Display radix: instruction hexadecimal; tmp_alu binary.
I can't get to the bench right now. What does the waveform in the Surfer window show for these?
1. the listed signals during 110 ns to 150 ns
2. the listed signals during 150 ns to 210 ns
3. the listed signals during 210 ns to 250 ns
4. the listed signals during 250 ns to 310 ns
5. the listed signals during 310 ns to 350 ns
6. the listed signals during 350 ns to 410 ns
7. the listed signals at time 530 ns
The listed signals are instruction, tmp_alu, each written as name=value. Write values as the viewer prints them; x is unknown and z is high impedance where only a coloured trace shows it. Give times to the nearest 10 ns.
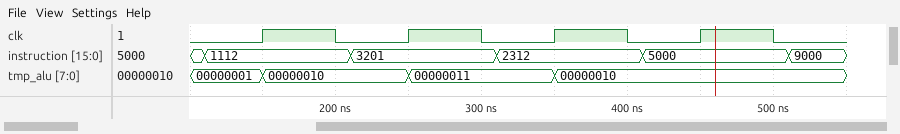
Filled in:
instruction=1112, tmp_alu=00000001
instruction=1112, tmp_alu=00000010
instruction=3201, tmp_alu=00000010
instruction=3201, tmp_alu=00000011
instruction=2312, tmp_alu=00000011
instruction=2312, tmp_alu=00000010
instruction=9000, tmp_alu=00000010
